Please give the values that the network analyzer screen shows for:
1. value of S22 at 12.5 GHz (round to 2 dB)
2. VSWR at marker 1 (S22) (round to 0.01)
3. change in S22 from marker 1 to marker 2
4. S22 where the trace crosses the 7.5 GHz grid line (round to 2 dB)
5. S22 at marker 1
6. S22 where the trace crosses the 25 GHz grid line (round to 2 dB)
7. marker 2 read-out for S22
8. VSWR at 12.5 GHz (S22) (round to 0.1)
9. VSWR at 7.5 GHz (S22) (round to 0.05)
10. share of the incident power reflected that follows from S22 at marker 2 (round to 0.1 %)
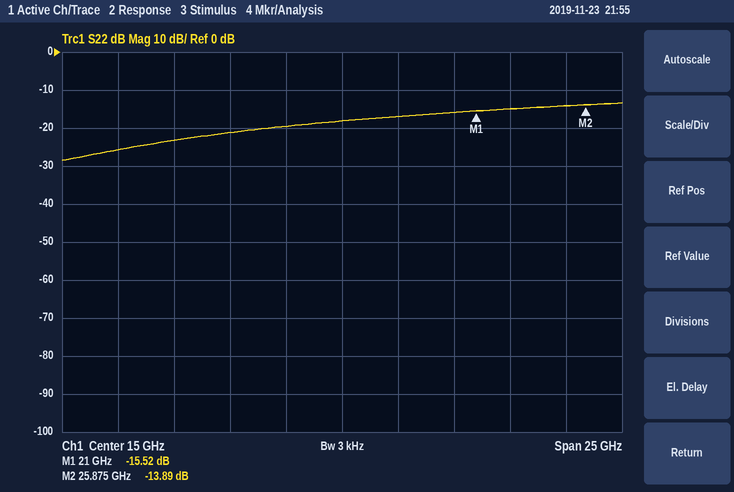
-20 dB
1.40
1.63 dB
-24 dB
-15.52 dB
-14 dB
-13.89 dB
1.2
1.15
4.1 %
